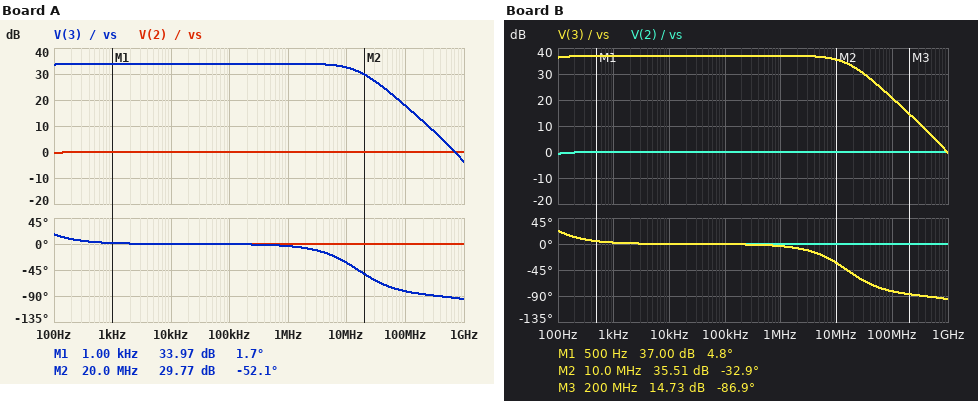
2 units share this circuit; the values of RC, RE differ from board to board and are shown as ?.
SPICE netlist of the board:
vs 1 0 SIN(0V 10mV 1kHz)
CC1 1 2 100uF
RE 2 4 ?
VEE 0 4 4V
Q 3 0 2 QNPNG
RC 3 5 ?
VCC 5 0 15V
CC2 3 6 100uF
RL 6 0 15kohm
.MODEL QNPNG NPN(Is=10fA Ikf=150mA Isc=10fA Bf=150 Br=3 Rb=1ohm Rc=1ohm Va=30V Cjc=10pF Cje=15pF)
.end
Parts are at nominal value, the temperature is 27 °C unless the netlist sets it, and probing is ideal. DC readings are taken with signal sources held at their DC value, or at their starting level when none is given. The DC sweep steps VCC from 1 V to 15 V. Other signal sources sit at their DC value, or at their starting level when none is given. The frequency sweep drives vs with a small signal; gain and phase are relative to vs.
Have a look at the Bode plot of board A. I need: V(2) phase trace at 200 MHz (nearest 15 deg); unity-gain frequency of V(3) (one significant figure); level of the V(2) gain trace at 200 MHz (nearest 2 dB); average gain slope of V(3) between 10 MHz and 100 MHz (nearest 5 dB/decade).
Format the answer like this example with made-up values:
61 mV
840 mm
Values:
0 deg
700 MHz
0 dB
-15 dB/decade
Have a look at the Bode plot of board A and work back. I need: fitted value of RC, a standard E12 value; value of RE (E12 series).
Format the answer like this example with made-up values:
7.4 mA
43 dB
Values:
3.3 kΩ
6.8 kΩ
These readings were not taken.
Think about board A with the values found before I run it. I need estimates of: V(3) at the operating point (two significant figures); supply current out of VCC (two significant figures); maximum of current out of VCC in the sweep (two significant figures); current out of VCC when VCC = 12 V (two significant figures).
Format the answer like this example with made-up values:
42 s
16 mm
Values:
13 V
490 µA
490 µA
490 µA
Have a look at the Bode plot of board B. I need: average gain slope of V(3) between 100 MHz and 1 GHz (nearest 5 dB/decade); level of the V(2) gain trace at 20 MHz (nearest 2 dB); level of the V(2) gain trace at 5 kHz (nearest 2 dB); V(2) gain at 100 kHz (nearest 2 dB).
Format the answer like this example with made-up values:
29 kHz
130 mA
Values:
-20 dB/decade
0 dB
0 dB
0 dB
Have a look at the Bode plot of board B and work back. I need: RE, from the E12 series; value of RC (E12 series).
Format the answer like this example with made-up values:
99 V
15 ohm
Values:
4.7 kΩ
3.3 kΩ
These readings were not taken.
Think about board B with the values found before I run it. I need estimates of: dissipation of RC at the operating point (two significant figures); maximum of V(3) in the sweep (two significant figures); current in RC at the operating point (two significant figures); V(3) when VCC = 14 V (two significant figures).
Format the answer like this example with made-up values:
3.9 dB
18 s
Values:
1.7 mW
13 V
710 µA
12 V
